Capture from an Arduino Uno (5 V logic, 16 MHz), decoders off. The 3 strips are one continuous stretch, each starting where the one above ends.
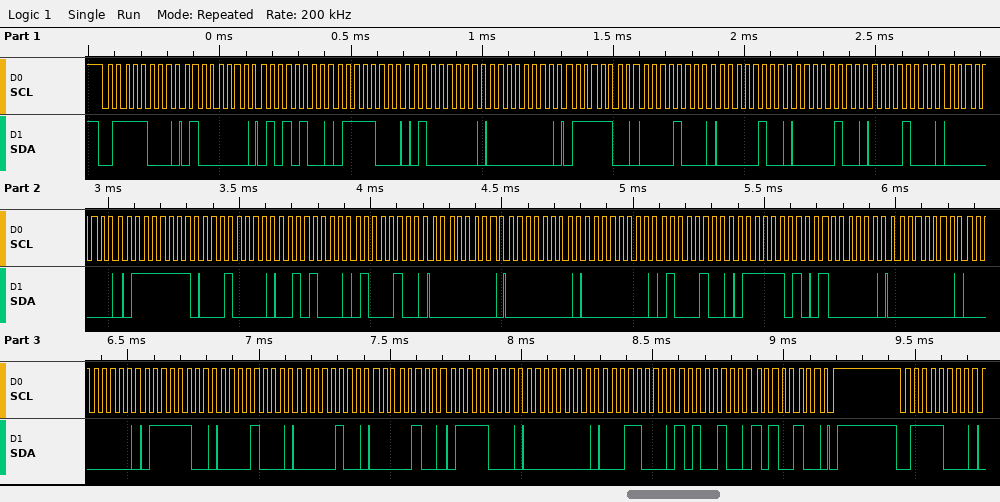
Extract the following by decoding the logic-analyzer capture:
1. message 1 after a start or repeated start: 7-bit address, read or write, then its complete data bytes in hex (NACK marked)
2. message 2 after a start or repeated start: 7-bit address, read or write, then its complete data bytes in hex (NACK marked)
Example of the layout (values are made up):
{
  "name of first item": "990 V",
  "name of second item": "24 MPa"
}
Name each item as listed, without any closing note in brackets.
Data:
{
  "message 1 after a start or repeated start: 7-bit address, read or write, then its complete data bytes in hex": "0x3C write: 40 54 78 40 00 7C 08 04 04 08 00 7F 10 28 44 00 00 00 44 7D 40 00 00 7C 08 04 04 78 00 18 A4 A4",
  "message 2 after a start or repeated start: 7-bit address, read or write, then its complete data bytes in hex": "0x3C write"
}
